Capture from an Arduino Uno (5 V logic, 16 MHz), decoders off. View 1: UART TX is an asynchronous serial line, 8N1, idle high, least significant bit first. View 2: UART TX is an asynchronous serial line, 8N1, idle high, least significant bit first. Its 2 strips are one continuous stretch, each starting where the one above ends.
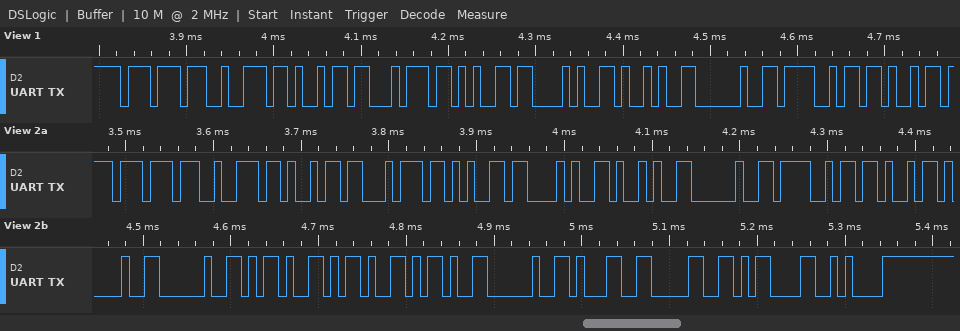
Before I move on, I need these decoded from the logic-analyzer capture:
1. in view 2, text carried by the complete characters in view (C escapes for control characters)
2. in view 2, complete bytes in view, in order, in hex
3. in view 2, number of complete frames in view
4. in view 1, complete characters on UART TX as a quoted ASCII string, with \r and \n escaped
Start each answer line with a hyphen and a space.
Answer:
- "write() OK! --- 10\r\n"
- 77 72 69 74 65 28 29 20 4F 4B 21 20 2D 2D 2D 20 31 30 0D 0A
- 20
- "write() OK"
